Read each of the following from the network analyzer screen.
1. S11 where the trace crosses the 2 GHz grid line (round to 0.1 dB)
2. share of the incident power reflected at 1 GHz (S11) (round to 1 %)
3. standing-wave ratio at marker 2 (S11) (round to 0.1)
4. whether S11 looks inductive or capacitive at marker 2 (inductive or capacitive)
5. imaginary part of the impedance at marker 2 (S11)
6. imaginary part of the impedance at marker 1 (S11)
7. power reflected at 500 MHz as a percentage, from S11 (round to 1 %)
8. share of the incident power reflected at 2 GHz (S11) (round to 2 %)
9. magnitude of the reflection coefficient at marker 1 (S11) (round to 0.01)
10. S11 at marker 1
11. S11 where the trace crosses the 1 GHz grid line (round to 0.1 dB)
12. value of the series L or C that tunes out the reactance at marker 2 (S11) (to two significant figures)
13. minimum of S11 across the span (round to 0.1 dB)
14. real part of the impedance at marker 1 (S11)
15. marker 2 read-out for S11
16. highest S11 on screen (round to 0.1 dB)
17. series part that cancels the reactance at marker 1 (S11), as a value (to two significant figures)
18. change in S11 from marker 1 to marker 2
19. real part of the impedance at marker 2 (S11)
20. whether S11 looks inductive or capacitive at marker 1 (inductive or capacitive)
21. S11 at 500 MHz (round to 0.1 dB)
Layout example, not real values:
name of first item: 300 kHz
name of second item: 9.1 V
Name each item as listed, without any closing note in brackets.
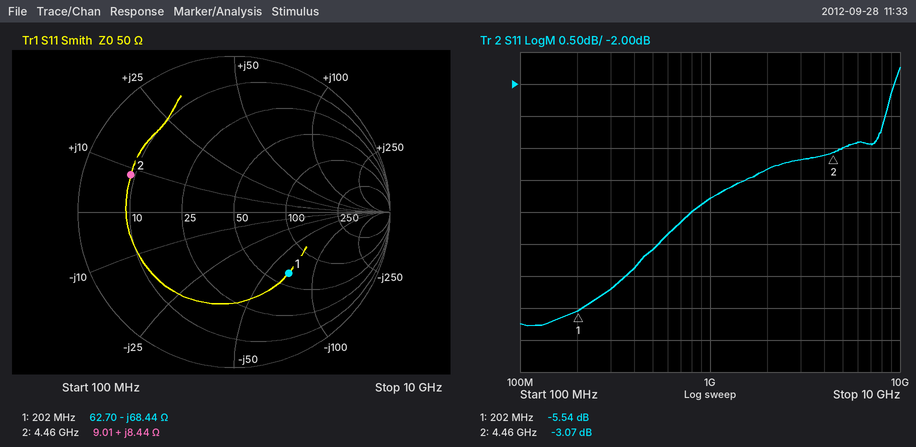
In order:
S11 where the trace crosses the 2 GHz grid line: -3.3 dB
share of the incident power reflected at 1 GHz (S11): 42 %
standing-wave ratio at marker 2 (S11): 5.7
whether S11 looks inductive or capacitive at marker 2: inductive
imaginary part of the impedance at marker 2: +8.44 Ω
imaginary part of the impedance at marker 1: -68.44 Ω
power reflected at 500 MHz as a percentage, from S11: 35 %
share of the incident power reflected at 2 GHz (S11): 46 %
magnitude of the reflection coefficient at marker 1 (S11): 0.53
S11 at marker 1: -5.54 dB
S11 where the trace crosses the 1 GHz grid line: -3.8 dB
value of the series L or C that tunes out the reactance at marker 2 (S11): 4.2 pF
minimum of S11 across the span: -5.8 dB
real part of the impedance at marker 1: 62.70 Ω
marker 2 read-out for S11: -3.07 dB
highest S11 on screen: -1.7 dB
series part that cancels the reactance at marker 1 (S11), as a value: 54 nH
change in S11 from marker 1 to marker 2: 2.47 dB
real part of the impedance at marker 2: 9.01 Ω
whether S11 looks inductive or capacitive at marker 1: capacitive
S11 at 500 MHz: -4.6 dB
